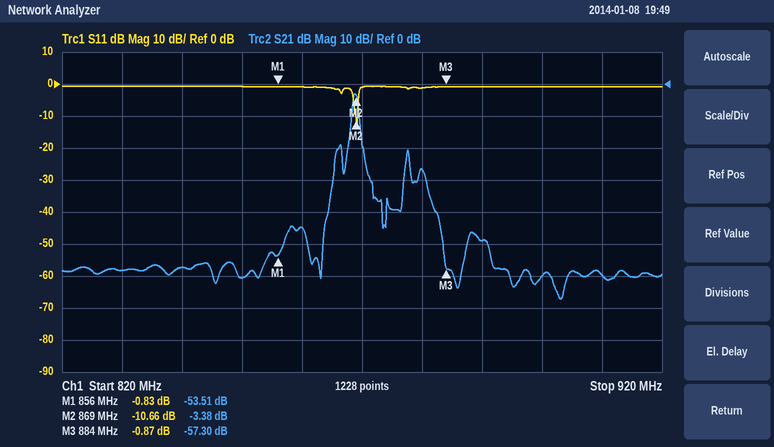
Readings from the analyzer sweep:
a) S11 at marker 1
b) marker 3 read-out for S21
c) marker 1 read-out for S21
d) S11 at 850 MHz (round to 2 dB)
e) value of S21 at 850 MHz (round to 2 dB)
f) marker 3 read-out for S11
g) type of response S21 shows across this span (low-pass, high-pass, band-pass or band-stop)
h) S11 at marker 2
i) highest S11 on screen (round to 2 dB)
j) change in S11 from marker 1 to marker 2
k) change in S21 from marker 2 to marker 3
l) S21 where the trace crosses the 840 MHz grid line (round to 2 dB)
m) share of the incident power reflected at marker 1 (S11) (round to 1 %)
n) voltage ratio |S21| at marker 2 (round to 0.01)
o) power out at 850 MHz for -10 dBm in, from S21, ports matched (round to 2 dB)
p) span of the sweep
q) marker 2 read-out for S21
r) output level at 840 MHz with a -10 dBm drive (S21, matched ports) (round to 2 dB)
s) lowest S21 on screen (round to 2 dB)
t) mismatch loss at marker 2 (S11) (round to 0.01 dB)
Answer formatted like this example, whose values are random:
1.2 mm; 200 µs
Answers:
-0.83 dB; -57.30 dB; -53.51 dB; 0 dB; -60 dB; -0.87 dB; band-pass; -10.66 dB; 0 dB; -9.83 dB; -53.92 dB; -58 dB; 83 %; 0.68; -70 dBm; 100 MHz; -3.38 dB; -68 dBm; -68 dB; 0.39 dB
